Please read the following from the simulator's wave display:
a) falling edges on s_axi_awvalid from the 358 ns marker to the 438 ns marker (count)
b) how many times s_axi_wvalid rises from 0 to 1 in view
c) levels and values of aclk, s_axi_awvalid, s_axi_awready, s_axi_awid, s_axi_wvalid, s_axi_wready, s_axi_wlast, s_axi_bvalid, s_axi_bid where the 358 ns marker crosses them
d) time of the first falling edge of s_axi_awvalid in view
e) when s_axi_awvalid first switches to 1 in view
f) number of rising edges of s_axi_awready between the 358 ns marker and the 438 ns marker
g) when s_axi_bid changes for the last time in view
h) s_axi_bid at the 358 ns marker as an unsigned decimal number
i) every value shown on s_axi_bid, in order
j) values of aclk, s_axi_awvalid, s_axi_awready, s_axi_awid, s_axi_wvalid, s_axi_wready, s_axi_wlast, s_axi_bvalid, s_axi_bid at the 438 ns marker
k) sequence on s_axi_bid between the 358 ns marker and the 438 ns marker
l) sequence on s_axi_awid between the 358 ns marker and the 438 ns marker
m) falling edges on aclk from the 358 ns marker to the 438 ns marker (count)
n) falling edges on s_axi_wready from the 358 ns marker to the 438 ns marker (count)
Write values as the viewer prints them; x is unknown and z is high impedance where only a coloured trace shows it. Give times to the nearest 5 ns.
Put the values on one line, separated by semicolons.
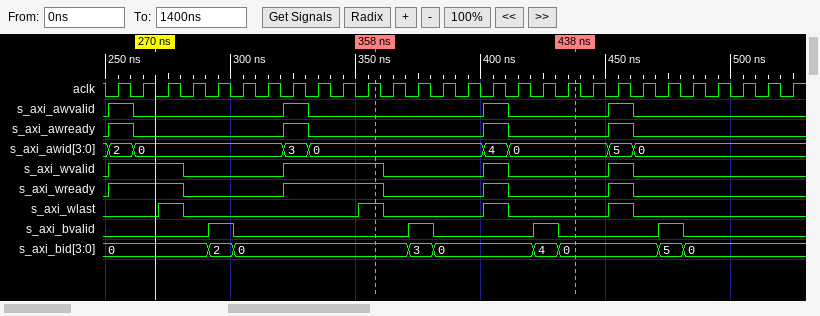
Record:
1; 4; aclk=1, s_axi_awvalid=0, s_axi_awready=0, s_axi_awid=0, s_axi_wvalid=1, s_axi_wready=1, s_axi_wlast=1, s_axi_bvalid=0, s_axi_bid=0; 260 ns; 250 ns; 1; 480 ns; 0; 0, 2, 0, 3, 0, 4, 0, 5, 0; aclk=1, s_axi_awvalid=0, s_axi_awready=0, s_axi_awid=0, s_axi_wvalid=0, s_axi_wready=0, s_axi_wlast=0, s_axi_bvalid=0, s_axi_bid=0; 0, 3, 0, 4, 0; 0, 4, 0; 8; 2
